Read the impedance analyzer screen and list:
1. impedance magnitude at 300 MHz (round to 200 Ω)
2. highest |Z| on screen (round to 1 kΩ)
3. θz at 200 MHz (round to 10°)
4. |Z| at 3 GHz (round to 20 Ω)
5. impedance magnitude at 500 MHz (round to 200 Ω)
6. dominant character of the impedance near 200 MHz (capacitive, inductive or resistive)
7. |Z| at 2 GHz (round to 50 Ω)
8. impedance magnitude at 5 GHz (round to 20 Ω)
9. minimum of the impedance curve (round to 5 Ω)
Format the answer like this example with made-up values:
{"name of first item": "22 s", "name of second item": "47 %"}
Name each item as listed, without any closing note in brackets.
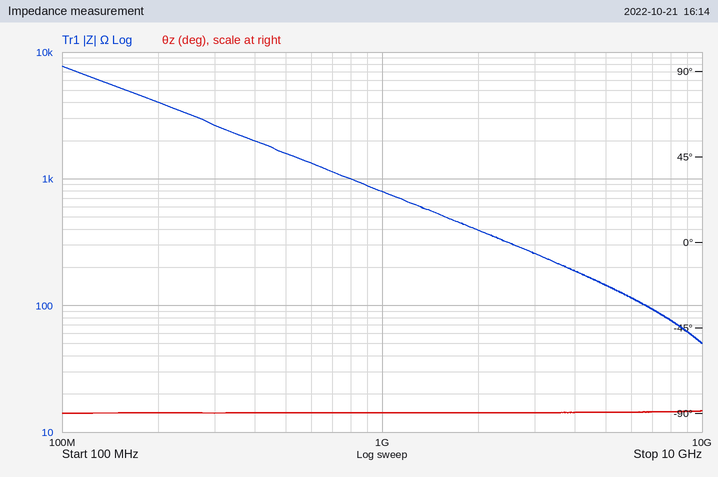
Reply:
{"impedance magnitude at 300 MHz": "2.6 kΩ", "highest |Z| on screen": "8 kΩ", "θz at 200 MHz": "-90°", "|Z| at 3 GHz": "260 Ω", "impedance magnitude at 500 MHz": "1.6 kΩ", "dominant character of the impedance near 200 MHz": "capacitive", "|Z| at 2 GHz": "400 Ω", "impedance magnitude at 5 GHz": "140 Ω", "minimum of the impedance curve": "50 Ω"}
